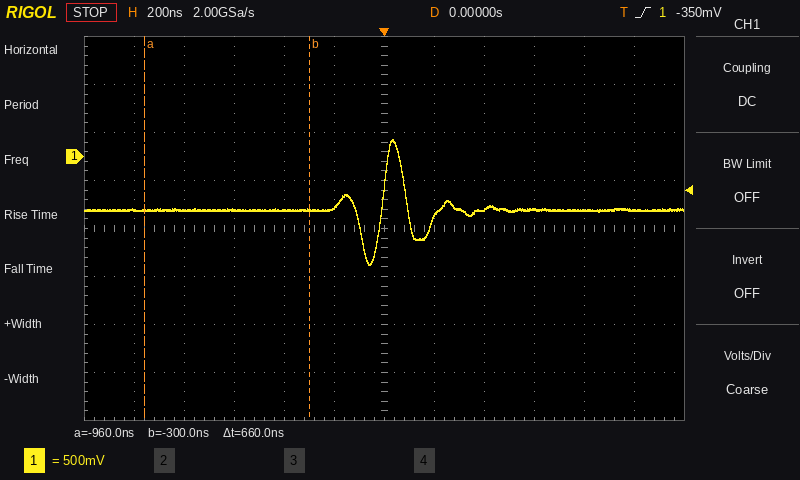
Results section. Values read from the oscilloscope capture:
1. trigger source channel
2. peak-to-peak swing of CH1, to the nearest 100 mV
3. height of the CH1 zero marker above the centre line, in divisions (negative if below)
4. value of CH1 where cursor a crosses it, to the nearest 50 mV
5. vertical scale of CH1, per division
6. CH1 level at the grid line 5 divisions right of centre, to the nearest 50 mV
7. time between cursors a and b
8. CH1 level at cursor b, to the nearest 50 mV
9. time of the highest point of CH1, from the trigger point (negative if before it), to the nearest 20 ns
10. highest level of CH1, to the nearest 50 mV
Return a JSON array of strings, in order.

["CH1", "1.30 V", "+1.5 div", "-550 mV", "500 mV", "-550 mV", "660 ns", "-550 mV", "+40 ns", "200 mV"]
